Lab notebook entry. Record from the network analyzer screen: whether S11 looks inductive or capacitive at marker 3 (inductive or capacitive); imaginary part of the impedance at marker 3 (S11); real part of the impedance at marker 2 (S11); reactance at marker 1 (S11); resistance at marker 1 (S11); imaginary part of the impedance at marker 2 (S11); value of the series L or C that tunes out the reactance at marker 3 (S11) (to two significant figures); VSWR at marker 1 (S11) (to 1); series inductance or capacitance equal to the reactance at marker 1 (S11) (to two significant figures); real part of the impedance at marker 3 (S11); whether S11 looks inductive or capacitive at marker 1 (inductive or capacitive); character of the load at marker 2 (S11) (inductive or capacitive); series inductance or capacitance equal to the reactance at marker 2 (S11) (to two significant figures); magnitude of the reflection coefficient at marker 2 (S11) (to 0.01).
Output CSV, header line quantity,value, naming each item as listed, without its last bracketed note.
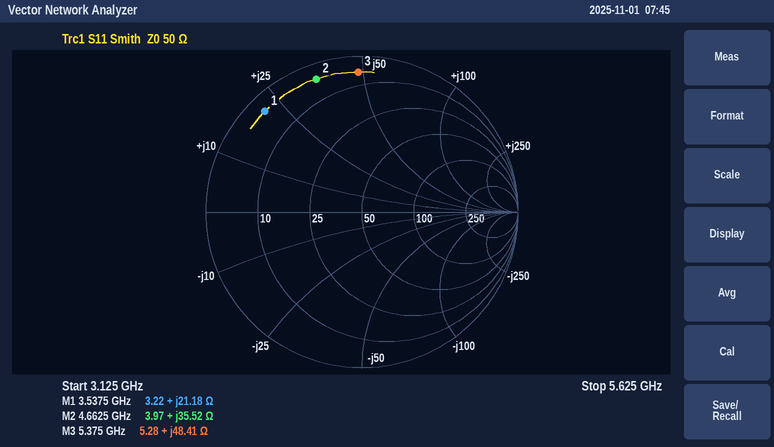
quantity,value
whether S11 looks inductive or capacitive at marker 3,inductive
imaginary part of the impedance at marker 3,+48.41 Ω
real part of the impedance at marker 2,3.97 Ω
reactance at marker 1,+21.18 Ω
resistance at marker 1,3.22 Ω
imaginary part of the impedance at marker 2,+35.52 Ω
value of the series L or C that tunes out the reactance at marker 3 (S11),610 fF
VSWR at marker 1 (S11),18
series inductance or capacitance equal to the reactance at marker 1 (S11),950 pH
real part of the impedance at marker 3,5.28 Ω
whether S11 looks inductive or capacitive at marker 1,inductive
character of the load at marker 2 (S11),inductive
series inductance or capacitance equal to the reactance at marker 2 (S11),1.2 nH
magnitude of the reflection coefficient at marker 2 (S11),0.90
